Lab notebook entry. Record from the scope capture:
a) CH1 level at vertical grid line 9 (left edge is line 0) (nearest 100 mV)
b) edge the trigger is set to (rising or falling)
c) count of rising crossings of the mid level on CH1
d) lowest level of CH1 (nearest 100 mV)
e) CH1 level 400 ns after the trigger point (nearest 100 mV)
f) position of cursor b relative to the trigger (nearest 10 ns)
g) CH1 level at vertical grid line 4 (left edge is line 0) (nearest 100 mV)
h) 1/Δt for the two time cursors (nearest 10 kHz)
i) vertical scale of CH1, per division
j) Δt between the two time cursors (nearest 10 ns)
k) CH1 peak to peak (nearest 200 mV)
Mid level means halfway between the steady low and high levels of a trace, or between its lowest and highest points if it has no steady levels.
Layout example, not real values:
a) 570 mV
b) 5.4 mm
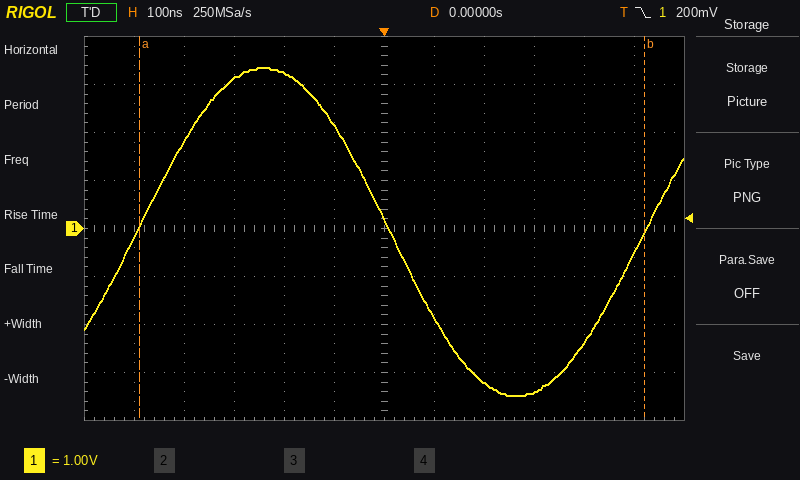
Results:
a) -3.4 V
b) falling
c) 2
d) -3.5 V
e) -2.4 V
f) +520 ns
g) 3.2 V
h) 990 kHz
i) 1 V
j) 1.01 µs
k) 6.8 V
